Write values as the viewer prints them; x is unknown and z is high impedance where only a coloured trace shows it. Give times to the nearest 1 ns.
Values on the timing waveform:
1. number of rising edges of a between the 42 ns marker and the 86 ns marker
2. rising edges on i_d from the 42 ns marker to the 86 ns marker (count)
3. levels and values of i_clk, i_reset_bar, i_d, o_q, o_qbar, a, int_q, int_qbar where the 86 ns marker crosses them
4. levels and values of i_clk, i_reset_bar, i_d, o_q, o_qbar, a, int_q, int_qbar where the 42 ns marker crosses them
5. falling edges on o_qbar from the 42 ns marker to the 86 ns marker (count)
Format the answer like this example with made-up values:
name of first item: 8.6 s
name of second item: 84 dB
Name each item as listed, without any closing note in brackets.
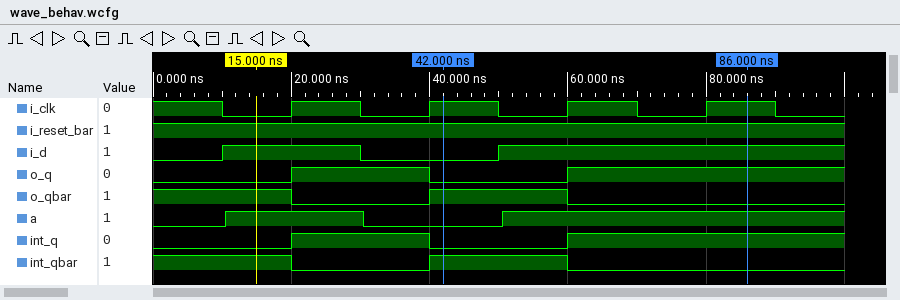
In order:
number of rising edges of a between the 42 ns marker and the 86 ns marker: 1
rising edges on i_d from the 42 ns marker to the 86 ns marker: 1
levels and values of i_clk, i_reset_bar, i_d, o_q, o_qbar, a, int_q, int_qbar where the 86 ns marker crosses them: i_clk=1, i_reset_bar=1, i_d=1, o_q=1, o_qbar=0, a=1, int_q=1, int_qbar=0
levels and values of i_clk, i_reset_bar, i_d, o_q, o_qbar, a, int_q, int_qbar where the 42 ns marker crosses them: i_clk=1, i_reset_bar=1, i_d=0, o_q=0, o_qbar=1, a=0, int_q=0, int_qbar=1
falling edges on o_qbar from the 42 ns marker to the 86 ns marker: 1
